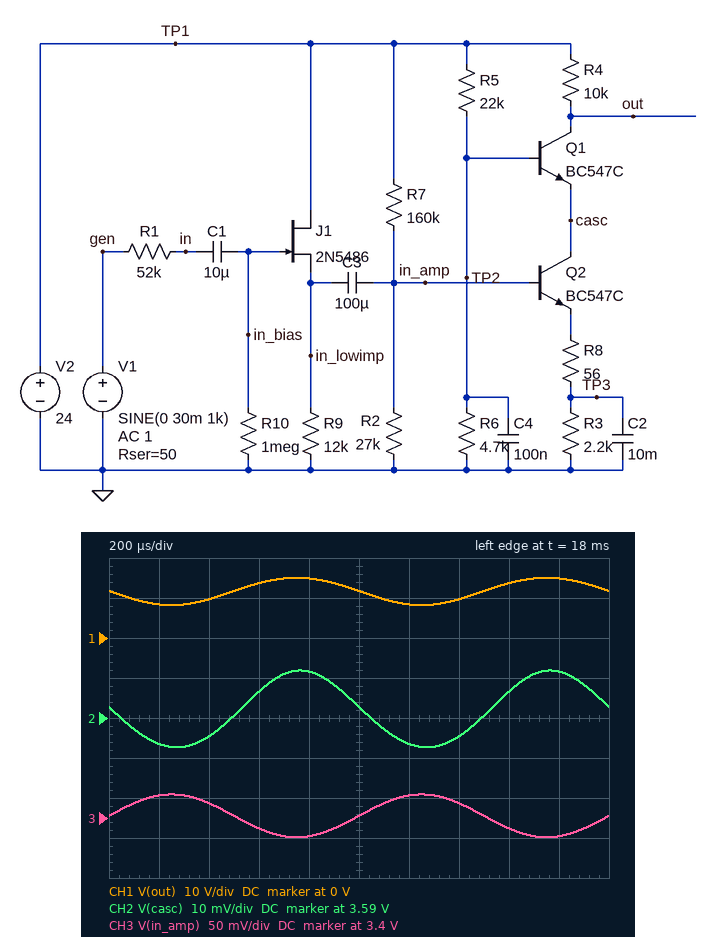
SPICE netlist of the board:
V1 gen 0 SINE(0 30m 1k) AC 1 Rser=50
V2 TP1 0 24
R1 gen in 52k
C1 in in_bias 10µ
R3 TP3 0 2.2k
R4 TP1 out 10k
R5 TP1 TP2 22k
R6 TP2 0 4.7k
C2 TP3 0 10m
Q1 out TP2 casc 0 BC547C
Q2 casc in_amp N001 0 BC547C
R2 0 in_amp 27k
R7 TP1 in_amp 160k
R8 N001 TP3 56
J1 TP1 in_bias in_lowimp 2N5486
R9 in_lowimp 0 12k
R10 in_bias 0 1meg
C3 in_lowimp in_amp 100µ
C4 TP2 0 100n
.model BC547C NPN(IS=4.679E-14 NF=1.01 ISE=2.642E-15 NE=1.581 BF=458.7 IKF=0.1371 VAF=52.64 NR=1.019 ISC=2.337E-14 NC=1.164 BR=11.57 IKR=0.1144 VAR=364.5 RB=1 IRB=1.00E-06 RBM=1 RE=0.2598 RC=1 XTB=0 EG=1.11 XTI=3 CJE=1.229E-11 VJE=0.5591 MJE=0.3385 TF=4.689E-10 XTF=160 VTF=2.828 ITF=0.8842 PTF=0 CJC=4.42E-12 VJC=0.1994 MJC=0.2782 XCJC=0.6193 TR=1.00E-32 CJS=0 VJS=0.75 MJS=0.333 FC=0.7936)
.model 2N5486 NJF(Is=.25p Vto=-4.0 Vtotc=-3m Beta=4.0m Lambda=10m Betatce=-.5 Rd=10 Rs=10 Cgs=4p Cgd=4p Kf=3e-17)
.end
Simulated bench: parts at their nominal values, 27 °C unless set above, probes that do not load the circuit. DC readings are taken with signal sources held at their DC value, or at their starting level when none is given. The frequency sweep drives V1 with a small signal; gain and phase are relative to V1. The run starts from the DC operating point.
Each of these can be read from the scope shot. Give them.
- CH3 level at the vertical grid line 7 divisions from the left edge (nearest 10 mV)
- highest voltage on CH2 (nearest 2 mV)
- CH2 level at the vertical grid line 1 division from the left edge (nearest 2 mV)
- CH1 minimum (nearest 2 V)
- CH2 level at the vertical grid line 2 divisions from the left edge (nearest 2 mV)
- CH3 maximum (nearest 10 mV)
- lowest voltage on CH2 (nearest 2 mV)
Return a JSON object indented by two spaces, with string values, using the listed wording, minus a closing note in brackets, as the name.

{
  "CH3 level at the vertical grid line 7 divisions from the left edge": "3.42 V",
  "highest voltage on CH2": "3.602 V",
  "CH2 level at the vertical grid line 1 division from the left edge": "3.584 V",
  "CH1 minimum": "8 V",
  "CH2 level at the vertical grid line 2 divisions from the left edge": "3.586 V",
  "CH3 maximum": "3.43 V",
  "lowest voltage on CH2": "3.582 V"
}
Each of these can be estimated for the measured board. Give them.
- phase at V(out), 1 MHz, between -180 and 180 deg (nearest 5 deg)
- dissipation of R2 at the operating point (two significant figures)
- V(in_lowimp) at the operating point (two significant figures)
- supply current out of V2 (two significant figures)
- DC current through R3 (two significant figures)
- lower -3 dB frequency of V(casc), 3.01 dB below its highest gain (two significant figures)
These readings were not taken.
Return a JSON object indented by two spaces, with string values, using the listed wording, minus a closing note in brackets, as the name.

{
  "phase at V(out), 1 MHz, between -180 and 180 deg": "155 deg",
  "dissipation of R2 at the operating point": "430 µW",
  "V(in_lowimp) at the operating point": "3.7 V",
  "supply current out of V2": "2.6 mA",
  "DC current through R3": "1.2 mA",
  "lower -3 dB frequency of V(casc), 3.01 dB below its highest gain": "280 mHz"
}
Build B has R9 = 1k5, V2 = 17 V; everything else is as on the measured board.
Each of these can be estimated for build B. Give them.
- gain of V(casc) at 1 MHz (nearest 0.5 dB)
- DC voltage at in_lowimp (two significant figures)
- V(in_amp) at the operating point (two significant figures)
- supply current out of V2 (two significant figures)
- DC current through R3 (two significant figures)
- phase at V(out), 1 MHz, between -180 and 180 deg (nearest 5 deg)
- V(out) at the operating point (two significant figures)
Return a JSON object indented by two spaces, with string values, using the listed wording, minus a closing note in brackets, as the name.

{
  "gain of V(casc) at 1 MHz": "-9.5 dB",
  "DC voltage at in_lowimp": "3.3 V",
  "V(in_amp) at the operating point": "2.4 V",
  "supply current out of V2": "3.7 mA",
  "DC current through R3": "800 µA",
  "phase at V(out), 1 MHz, between -180 and 180 deg": "150 deg",
  "V(out) at the operating point": "9.1 V"
}
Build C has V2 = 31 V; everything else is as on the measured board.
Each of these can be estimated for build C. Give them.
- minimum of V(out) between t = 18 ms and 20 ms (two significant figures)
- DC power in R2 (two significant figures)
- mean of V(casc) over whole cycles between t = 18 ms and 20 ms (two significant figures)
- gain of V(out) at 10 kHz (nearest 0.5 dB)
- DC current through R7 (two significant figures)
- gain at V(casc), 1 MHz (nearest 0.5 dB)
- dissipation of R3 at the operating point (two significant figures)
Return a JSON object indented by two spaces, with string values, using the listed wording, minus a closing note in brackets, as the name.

{
  "minimum of V(out) between t = 18 ms and 20 ms": "11 V",
  "DC power in R2": "710 µW",
  "mean of V(casc) over whole cycles between t = 18 ms and 20 ms": "4.8 V",
  "gain of V(out) at 10 kHz": "42.0 dB",
  "DC current through R7": "170 µA",
  "gain at V(casc), 1 MHz": "-12.0 dB",
  "dissipation of R3 at the operating point": "6.1 mW"
}
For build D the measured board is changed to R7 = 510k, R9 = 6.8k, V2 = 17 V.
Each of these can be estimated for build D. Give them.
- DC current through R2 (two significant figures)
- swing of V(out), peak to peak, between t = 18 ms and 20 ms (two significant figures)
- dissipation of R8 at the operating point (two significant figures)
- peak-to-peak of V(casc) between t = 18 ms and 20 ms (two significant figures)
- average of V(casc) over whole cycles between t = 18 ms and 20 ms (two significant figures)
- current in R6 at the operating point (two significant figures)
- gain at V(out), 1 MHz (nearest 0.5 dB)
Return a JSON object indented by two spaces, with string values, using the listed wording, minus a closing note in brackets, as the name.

{
  "DC current through R2": "31 µA",
  "swing of V(out), peak to peak, between t = 18 ms and 20 ms": "2.1 V",
  "dissipation of R8 at the operating point": "870 nW",
  "peak-to-peak of V(casc) between t = 18 ms and 20 ms": "43 mV",
  "average of V(casc) over whole cycles between t = 18 ms and 20 ms": "2.4 V",
  "current in R6 at the operating point": "640 µA",
  "gain at V(out), 1 MHz": "30.0 dB"
}
